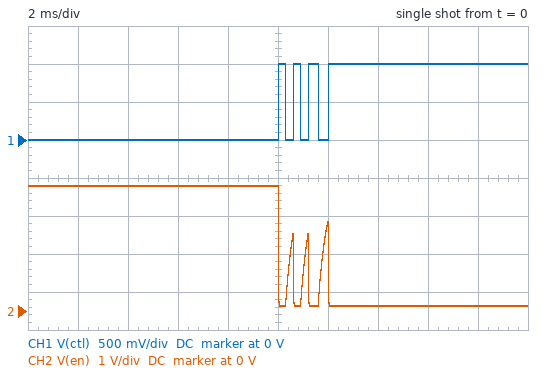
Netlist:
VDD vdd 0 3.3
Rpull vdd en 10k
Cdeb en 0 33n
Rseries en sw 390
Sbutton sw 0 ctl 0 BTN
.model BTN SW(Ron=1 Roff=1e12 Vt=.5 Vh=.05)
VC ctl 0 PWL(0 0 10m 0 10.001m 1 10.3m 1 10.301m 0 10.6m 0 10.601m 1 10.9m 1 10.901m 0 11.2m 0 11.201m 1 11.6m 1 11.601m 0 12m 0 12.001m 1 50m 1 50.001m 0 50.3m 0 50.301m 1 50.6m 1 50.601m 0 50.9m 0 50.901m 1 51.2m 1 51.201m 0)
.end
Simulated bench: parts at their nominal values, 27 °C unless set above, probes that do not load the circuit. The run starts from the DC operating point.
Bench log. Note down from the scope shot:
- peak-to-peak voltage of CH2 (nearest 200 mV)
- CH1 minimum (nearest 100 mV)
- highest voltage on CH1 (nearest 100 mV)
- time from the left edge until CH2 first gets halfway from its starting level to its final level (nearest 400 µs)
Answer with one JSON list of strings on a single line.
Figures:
["3.2 V", "0 V", "1.0 V", "10.0 ms"]
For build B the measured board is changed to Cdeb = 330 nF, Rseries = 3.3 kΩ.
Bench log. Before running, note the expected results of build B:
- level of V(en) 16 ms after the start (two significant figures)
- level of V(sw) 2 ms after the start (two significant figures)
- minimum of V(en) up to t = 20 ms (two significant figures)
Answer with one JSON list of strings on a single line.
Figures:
["830 mV", "3.3 V", "820 mV"]
